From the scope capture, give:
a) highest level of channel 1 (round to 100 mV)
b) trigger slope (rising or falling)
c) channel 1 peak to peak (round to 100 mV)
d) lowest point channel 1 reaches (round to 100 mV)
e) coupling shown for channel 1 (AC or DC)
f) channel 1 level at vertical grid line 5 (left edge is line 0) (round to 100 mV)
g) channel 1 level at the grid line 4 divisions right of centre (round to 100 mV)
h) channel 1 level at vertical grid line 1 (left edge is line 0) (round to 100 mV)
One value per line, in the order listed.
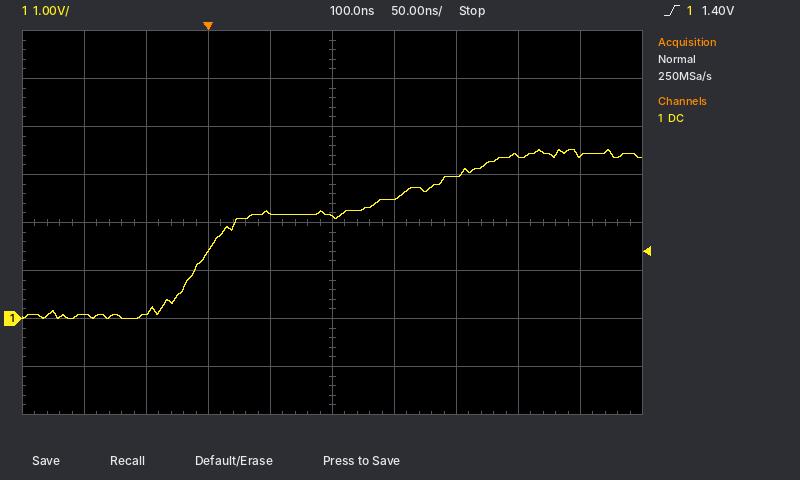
3.5 V
rising
3.5 V
0.0 V
DC
2.1 V
3.4 V
100 mV
